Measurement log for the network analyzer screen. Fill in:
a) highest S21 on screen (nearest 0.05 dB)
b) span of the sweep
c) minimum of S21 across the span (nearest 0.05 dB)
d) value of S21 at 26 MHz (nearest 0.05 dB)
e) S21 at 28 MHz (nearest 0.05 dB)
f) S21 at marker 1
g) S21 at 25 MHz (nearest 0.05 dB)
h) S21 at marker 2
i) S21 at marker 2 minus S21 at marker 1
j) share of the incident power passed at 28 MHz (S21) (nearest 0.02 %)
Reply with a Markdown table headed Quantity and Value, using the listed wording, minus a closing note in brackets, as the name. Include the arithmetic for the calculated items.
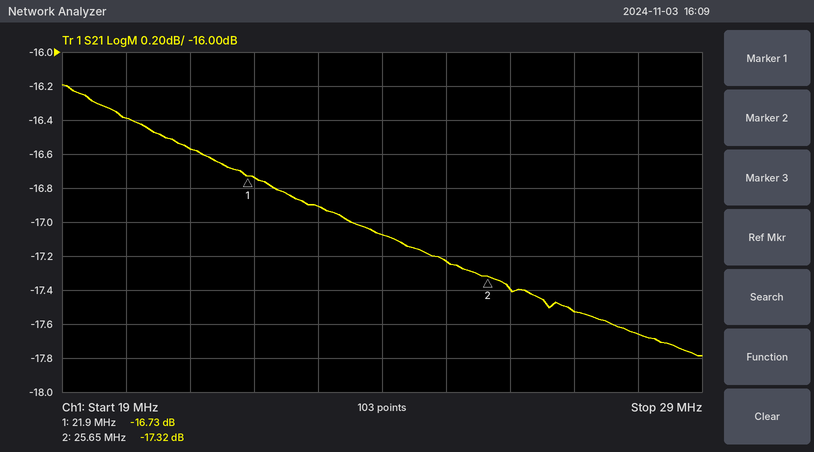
| Quantity | Value |
|---|---|
| highest S21 on screen | -16.20 dB |
| span of the sweep | 10 MHz |
| minimum of S21 across the span | -17.80 dB |
| value of S21 at 26 MHz | -17.40 dB |
| S21 at 28 MHz | -17.65 dB |
| S21 at marker 1 | -16.73 dB |
| S21 at 25 MHz | -17.25 dB |
| S21 at marker 2 | -17.32 dB |
| S21 at marker 2 minus S21 at marker 1 | -17.32 − (-16.73) = -0.59 dB |
| share of the incident power passed at 28 MHz (S21) | 10^(-17.65/10) ≈ 1.72 % |
